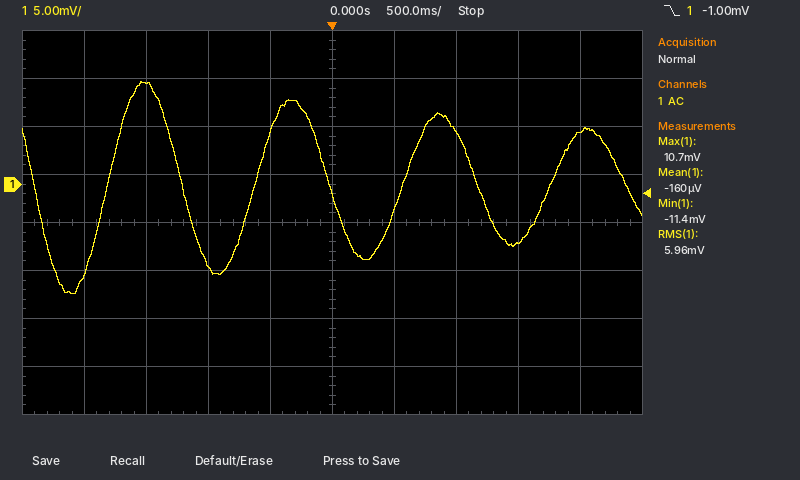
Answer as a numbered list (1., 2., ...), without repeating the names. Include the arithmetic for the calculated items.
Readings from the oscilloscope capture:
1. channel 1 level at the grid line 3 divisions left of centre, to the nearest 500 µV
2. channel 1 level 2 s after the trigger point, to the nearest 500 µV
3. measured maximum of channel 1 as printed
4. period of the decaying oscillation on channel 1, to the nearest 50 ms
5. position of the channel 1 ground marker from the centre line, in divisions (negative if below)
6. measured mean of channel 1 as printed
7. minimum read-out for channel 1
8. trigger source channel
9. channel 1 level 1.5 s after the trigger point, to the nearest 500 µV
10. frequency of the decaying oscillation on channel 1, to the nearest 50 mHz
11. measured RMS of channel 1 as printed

1. 10.5 mV
2. 5.5 mV
3. 10.7 mV
4. 1.20 s
5. +0.8 div
6. -160 µV
7. -11.4 mV
8. channel 1
9. -6.0 mV
10. 1 / 1.20 s ≈ 833 mHz, so 850 mHz to the nearest 50 mHz
11. 5.96 mV
